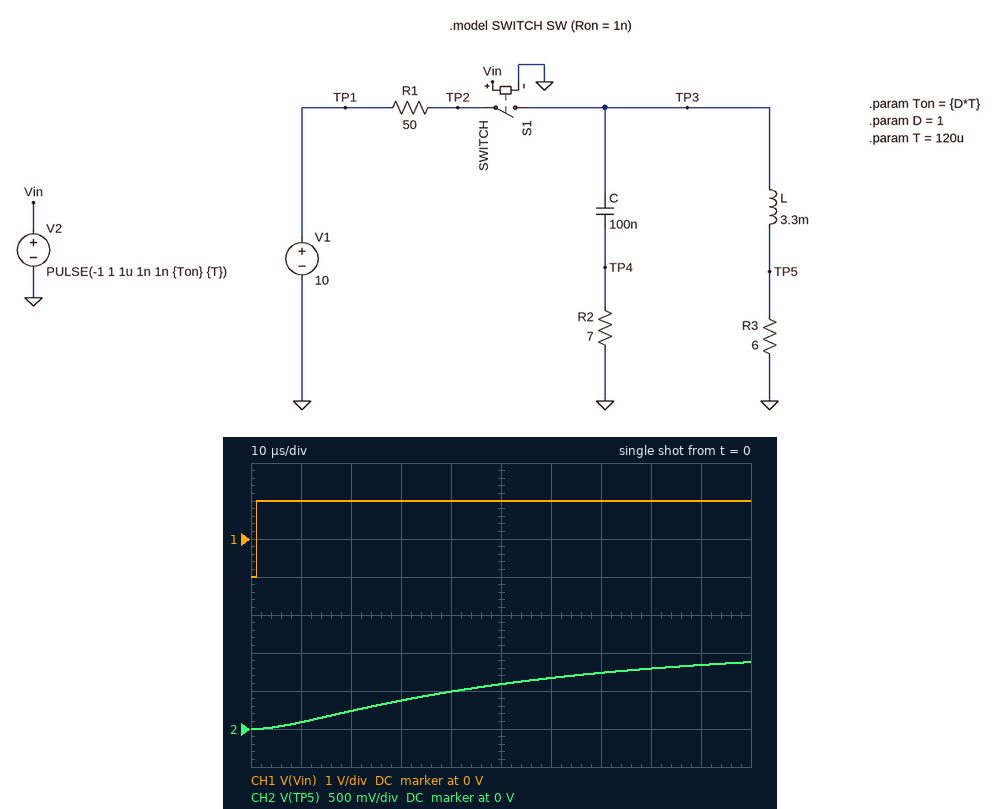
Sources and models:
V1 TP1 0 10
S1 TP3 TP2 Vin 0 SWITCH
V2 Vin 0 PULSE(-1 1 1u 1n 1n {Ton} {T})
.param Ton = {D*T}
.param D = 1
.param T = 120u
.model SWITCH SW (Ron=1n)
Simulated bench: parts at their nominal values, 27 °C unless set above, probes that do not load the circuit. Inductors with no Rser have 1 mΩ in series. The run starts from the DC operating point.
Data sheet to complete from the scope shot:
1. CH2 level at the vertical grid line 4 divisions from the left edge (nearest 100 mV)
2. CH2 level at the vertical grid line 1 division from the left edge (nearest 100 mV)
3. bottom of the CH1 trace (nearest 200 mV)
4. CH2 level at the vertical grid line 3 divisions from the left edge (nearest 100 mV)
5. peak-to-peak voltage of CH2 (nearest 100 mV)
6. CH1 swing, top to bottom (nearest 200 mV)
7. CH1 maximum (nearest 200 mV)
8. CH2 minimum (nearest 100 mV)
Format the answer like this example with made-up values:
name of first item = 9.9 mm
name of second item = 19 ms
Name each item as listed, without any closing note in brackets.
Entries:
CH2 level at the vertical grid line 4 divisions from the left edge = 500 mV
CH2 level at the vertical grid line 1 division from the left edge = 100 mV
bottom of the CH1 trace = -1.0 V
CH2 level at the vertical grid line 3 divisions from the left edge = 400 mV
peak-to-peak voltage of CH2 = 900 mV
CH1 swing, top to bottom = 2.0 V
CH1 maximum = 1.0 V
CH2 minimum = 0 V
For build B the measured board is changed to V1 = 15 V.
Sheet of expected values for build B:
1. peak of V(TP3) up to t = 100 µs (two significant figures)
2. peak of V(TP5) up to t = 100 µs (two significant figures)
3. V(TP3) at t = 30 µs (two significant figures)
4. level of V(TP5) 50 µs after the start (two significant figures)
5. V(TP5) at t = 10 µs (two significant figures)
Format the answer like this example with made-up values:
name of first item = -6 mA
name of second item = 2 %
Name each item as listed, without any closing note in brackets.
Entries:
peak of V(TP3) up to t = 100 µs = 13 V
peak of V(TP5) up to t = 100 µs = 1.3 V
V(TP3) at t = 30 µs = 11 V
level of V(TP5) 50 µs after the start = 880 mV
V(TP5) at t = 10 µs = 130 mV
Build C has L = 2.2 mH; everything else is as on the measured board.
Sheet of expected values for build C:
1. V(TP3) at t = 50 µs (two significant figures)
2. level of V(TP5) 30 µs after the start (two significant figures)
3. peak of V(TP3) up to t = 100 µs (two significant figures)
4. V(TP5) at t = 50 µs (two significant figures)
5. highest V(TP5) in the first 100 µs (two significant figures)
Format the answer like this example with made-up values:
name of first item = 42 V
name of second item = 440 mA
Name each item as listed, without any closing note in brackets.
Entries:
V(TP3) at t = 50 µs = 4.1 V
level of V(TP5) 30 µs after the start = 520 mV
peak of V(TP3) up to t = 100 µs = 8.0 V
V(TP5) at t = 50 µs = 760 mV
highest V(TP5) in the first 100 µs = 1.0 V
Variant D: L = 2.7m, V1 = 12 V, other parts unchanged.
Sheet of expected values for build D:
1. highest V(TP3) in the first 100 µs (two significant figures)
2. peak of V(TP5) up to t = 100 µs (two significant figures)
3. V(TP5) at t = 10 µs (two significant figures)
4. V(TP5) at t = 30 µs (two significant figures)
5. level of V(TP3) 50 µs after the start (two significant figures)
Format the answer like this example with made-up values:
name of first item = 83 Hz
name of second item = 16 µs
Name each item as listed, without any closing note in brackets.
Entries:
highest V(TP3) in the first 100 µs = 9.9 V
peak of V(TP5) up to t = 100 µs = 1.1 V
V(TP5) at t = 10 µs = 130 mV
V(TP5) at t = 30 µs = 530 mV
level of V(TP3) 50 µs after the start = 5.8 V
